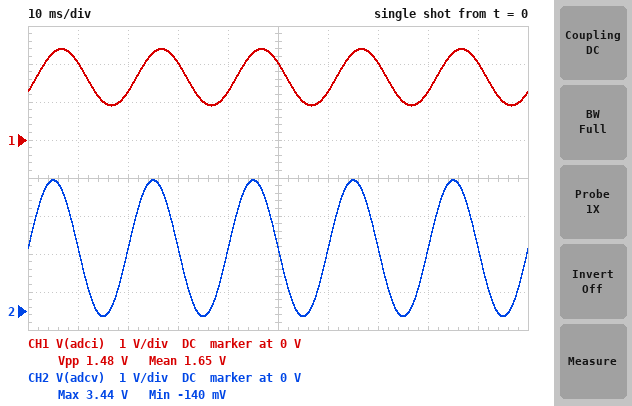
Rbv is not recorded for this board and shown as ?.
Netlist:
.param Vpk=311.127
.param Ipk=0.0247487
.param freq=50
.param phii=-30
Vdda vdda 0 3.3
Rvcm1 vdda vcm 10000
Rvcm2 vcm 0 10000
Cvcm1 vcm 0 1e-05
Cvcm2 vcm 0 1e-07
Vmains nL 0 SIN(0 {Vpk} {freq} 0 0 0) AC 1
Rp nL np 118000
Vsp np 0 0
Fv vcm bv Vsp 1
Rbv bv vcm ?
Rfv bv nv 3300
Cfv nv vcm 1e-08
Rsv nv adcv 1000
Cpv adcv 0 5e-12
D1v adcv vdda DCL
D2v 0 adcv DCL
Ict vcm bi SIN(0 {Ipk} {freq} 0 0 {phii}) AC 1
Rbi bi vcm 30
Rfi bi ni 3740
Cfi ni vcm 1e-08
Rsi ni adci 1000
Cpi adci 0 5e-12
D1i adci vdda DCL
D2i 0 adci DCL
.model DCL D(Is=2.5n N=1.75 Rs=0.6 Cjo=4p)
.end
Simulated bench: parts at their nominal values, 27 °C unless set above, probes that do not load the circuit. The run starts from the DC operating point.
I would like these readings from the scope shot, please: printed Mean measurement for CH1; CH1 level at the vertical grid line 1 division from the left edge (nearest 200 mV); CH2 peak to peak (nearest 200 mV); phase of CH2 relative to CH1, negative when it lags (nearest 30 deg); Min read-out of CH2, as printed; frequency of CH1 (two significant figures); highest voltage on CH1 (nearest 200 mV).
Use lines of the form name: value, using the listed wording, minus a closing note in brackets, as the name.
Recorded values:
printed Mean measurement for CH1: 1.65 V
CH1 level at the vertical grid line 1 division from the left edge: 2.0 V
CH2 peak to peak: 3.6 V
phase of CH2 relative to CH1, negative when it lags: 30 deg
Min read-out of CH2, as printed: -140 mV
frequency of CH1: 50 Hz
highest voltage on CH1: 2.4 V
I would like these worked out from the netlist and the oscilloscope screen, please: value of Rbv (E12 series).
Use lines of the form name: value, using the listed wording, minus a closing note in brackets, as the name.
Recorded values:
value of Rbv: 680 Ω
